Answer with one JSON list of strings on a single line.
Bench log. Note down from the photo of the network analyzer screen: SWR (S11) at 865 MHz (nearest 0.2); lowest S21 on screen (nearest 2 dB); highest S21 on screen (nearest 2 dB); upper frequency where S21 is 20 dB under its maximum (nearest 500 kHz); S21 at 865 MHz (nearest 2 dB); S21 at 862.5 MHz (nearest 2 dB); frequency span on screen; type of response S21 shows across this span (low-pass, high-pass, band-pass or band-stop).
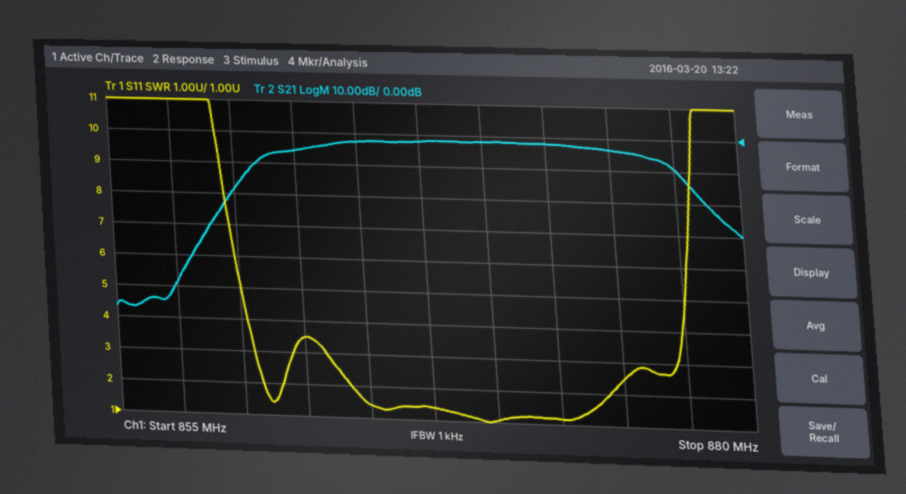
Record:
["1.4", "-56 dB", "-2 dB", "879.0 MHz", "-2 dB", "-6 dB", "25 MHz", "band-pass"]
